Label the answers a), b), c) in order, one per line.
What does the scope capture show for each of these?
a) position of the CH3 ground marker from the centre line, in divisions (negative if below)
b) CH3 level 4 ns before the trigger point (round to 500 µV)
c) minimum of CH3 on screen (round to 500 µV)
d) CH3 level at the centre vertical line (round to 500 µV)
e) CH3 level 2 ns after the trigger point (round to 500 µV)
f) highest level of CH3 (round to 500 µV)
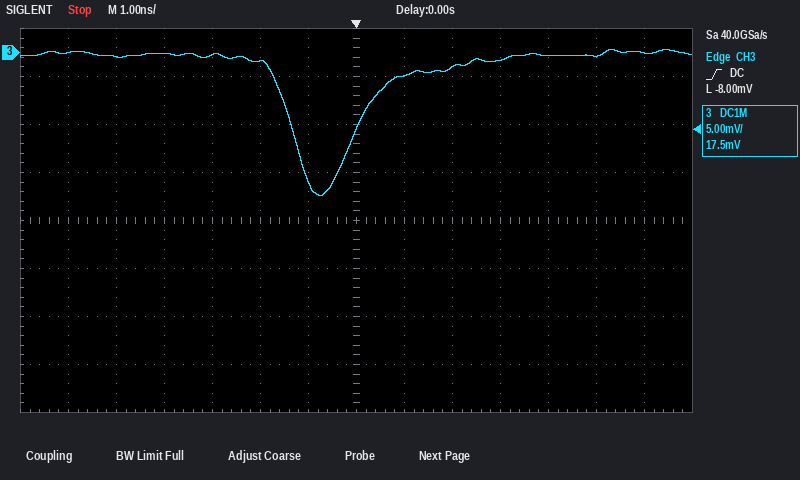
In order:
a) +3.5 div
b) 0.0 mV
c) -15.0 mV
d) -8.0 mV
e) -1.5 mV
f) 500 µV
